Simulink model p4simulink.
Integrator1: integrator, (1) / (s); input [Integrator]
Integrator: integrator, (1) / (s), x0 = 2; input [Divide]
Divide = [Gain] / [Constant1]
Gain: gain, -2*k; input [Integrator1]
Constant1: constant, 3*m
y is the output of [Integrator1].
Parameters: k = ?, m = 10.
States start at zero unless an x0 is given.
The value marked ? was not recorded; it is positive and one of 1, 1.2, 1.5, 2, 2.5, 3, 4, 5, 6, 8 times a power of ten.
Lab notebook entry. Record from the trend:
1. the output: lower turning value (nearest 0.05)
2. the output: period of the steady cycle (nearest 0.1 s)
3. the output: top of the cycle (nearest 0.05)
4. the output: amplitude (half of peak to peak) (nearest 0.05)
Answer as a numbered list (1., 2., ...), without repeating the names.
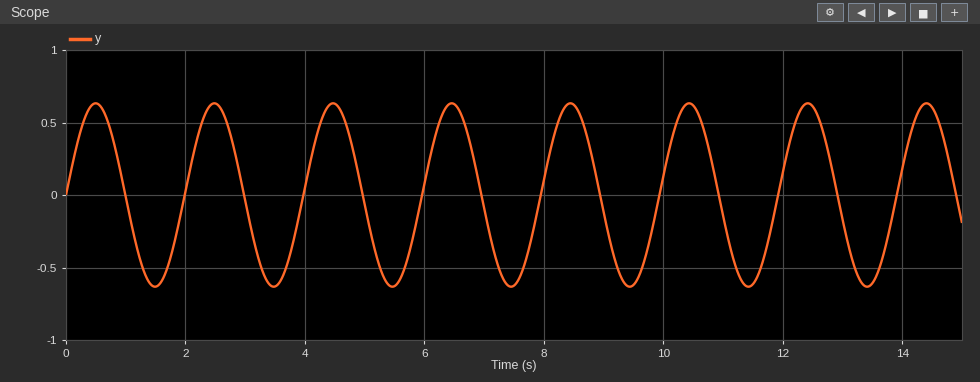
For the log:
1. -0.65
2. 2.0 s
3. 0.65
4. 0.65
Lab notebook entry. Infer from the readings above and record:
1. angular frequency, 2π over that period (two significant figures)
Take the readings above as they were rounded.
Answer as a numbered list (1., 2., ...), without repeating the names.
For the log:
1. 3.1 rad/s
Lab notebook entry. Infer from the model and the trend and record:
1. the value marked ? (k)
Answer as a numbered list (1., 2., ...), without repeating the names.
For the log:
1. 150
